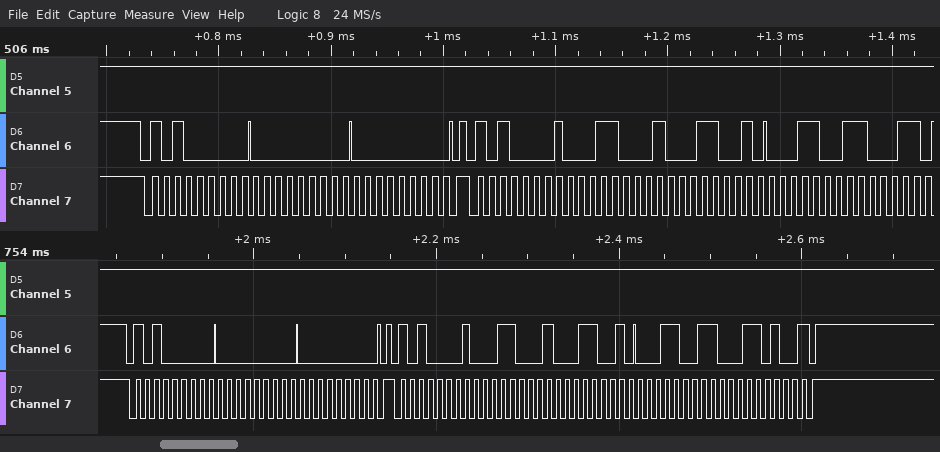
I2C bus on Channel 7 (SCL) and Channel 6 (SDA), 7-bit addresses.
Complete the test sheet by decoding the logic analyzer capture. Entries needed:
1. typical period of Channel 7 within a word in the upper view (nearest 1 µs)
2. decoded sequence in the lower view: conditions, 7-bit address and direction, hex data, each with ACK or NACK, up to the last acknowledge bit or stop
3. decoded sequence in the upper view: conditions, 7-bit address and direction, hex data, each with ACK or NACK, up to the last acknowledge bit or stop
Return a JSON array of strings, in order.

["10 µs", "start, address 50 write ACK, 00 ACK, 00 ACK, stop, start, address 50 read ACK, 31 ACK, 32 ACK, 33 ACK, 34 NACK, stop", "start, address 50 write ACK, 00 ACK, 00 ACK, stop, start, address 50 read ACK, 31 ACK, 32 ACK, 33 ACK"]
